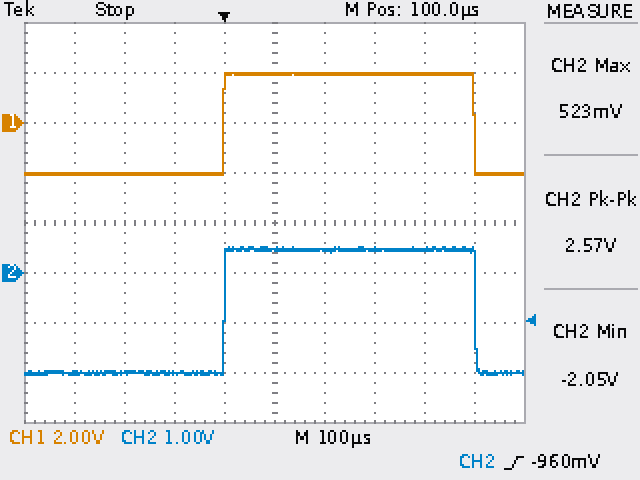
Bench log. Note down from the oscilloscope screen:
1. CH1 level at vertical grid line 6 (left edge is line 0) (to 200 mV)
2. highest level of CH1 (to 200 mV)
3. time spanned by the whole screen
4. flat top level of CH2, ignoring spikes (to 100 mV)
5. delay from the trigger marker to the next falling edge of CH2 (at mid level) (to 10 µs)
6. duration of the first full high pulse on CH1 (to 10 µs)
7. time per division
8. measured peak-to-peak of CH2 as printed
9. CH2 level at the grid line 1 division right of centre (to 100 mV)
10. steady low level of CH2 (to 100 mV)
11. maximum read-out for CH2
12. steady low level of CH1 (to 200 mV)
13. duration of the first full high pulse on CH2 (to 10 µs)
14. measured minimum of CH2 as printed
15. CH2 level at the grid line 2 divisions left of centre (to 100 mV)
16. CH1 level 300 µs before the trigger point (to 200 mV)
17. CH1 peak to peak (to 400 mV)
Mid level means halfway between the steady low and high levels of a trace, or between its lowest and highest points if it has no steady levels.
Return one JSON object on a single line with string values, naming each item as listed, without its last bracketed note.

{"CH1 level at vertical grid line 6 (left edge is line 0)": "2.0 V", "highest level of CH1": "2.0 V", "time spanned by the whole screen": "1 ms", "flat top level of CH2, ignoring spikes": "500 mV", "delay from the trigger marker to the next falling edge of CH2 (at mid level)": "500 µs", "duration of the first full high pulse on CH1": "500 µs", "time per division": "100 µs", "measured peak-to-peak of CH2 as printed": "2.57 V", "CH2 level at the grid line 1 division right of centre": "500 mV", "steady low level of CH2": "-2.0 V", "maximum read-out for CH2": "523 mV", "steady low level of CH1": "-2.0 V", "duration of the first full high pulse on CH2": "500 µs", "measured minimum of CH2 as printed": "-2.05 V", "CH2 level at the grid line 2 divisions left of centre": "-2.0 V", "CH1 level 300 µs before the trigger point": "-2.0 V", "CH1 peak to peak": "4.0 V"}
